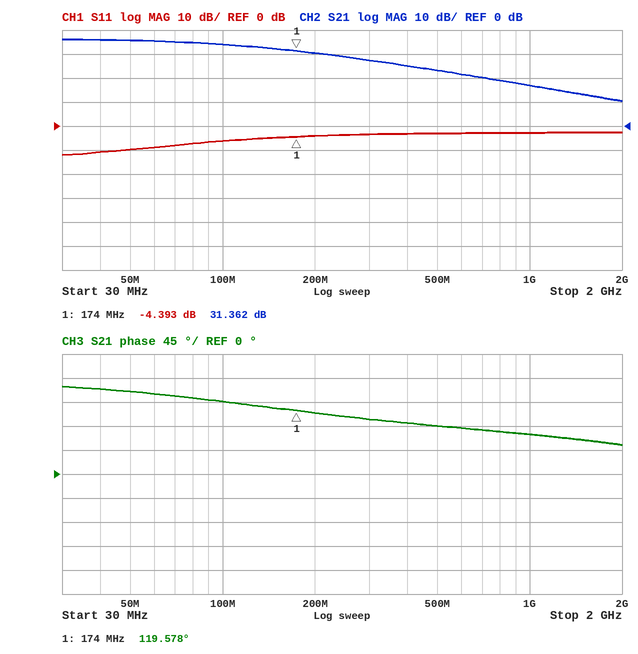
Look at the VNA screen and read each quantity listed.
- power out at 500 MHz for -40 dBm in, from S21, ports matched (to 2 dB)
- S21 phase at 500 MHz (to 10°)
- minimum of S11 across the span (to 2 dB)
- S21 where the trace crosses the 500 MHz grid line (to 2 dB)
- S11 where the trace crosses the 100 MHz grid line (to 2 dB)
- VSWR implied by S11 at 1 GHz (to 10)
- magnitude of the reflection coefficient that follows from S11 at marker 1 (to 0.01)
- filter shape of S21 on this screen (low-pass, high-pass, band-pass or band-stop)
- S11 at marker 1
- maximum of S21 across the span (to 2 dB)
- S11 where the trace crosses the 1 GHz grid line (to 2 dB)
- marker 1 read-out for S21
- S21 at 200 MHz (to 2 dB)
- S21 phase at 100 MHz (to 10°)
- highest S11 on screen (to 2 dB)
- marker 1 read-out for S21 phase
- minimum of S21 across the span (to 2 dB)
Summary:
-16 dBm
90°
-12 dB
24 dB
-6 dB
10
0.60
low-pass
-4.393 dB
36 dB
-2 dB
31.362 dB
30 dB
140°
-2 dB
119.578°
10 dB
